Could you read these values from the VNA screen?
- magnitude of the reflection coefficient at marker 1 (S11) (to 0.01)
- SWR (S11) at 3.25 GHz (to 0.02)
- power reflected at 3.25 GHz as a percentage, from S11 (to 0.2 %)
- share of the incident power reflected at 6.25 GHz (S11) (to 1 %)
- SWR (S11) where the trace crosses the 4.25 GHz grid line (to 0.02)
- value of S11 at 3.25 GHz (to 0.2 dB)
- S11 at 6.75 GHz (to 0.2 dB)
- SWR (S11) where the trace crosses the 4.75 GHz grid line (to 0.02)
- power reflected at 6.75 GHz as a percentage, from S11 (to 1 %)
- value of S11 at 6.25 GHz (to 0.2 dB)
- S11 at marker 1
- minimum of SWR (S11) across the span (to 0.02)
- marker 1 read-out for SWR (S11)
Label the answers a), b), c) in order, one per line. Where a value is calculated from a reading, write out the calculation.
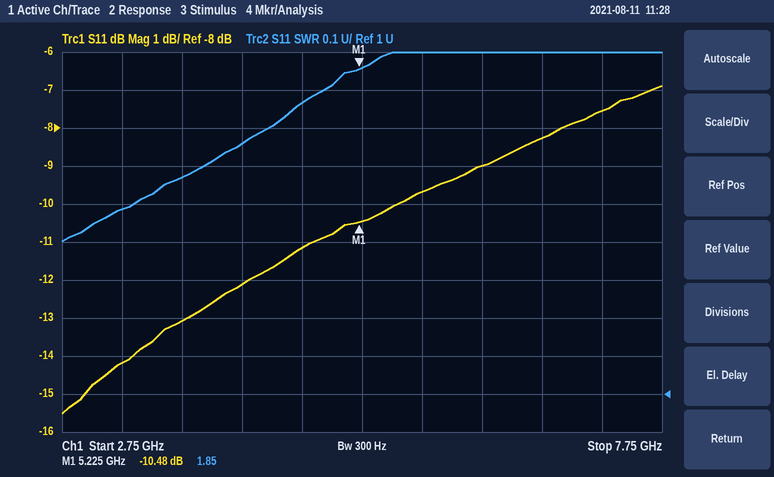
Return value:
a) 10^(-10.48/20) ≈ 0.30
b) 1.48
c) 10^(-14.2/10) ≈ 3.8 %
d) 10^(-9/10) ≈ 13 %
e) 1.66
f) -14.2 dB
g) -8.2 dB
h) 1.76
i) 10^(-8.2/10) ≈ 15 %
j) -9.0 dB
k) -10.48 dB
l) 1.40
m) 1.85
